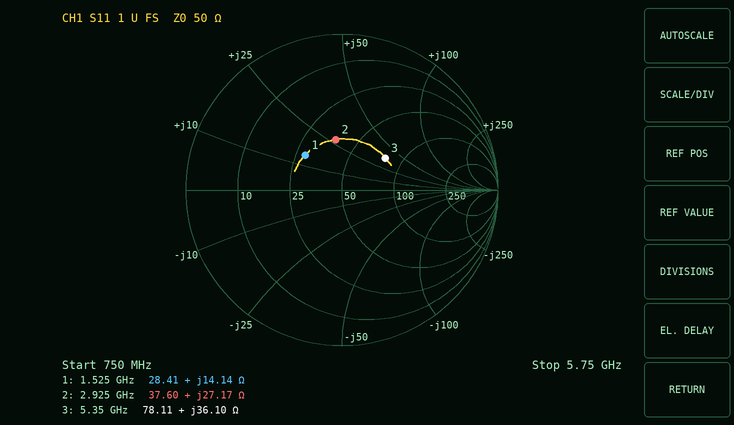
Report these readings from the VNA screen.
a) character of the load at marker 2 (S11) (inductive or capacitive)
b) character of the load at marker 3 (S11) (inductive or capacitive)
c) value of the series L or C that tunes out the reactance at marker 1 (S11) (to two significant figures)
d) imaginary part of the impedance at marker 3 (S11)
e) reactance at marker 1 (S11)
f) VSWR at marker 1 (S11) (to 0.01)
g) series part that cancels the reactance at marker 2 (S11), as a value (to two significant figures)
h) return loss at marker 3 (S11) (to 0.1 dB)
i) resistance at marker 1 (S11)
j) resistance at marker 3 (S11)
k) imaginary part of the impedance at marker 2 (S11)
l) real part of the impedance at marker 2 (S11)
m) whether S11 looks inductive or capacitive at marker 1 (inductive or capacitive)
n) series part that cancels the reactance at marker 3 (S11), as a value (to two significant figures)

inductive
inductive
7.4 pF
+36.10 Ω
+14.14 Ω
1.96
2.0 pF
9.3 dB
28.41 Ω
78.11 Ω
+27.17 Ω
37.60 Ω
inductive
820 fF
